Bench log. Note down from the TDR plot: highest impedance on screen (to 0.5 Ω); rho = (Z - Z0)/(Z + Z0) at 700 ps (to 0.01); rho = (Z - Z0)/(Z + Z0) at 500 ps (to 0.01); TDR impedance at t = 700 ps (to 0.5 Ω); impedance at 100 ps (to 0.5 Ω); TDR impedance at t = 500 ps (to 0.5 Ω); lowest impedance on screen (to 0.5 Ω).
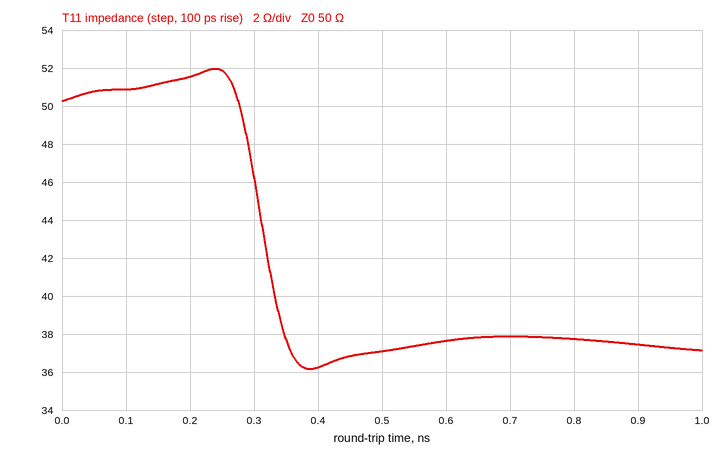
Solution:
52.0 Ω
-0.14
-0.15
38.0 Ω
51.0 Ω
37.0 Ω
36.0 Ω
